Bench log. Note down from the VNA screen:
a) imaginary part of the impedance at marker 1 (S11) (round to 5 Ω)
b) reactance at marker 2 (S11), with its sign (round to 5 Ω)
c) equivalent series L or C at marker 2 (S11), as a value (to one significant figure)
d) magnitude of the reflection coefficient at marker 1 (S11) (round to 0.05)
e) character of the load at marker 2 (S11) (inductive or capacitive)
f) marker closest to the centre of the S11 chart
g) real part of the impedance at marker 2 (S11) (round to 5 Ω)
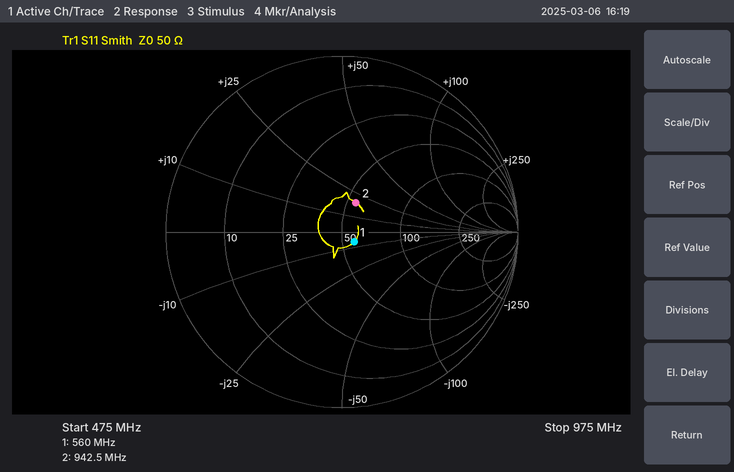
-5 Ω
+20 Ω
3 nH
0.10
inductive
marker 1
55 Ω
